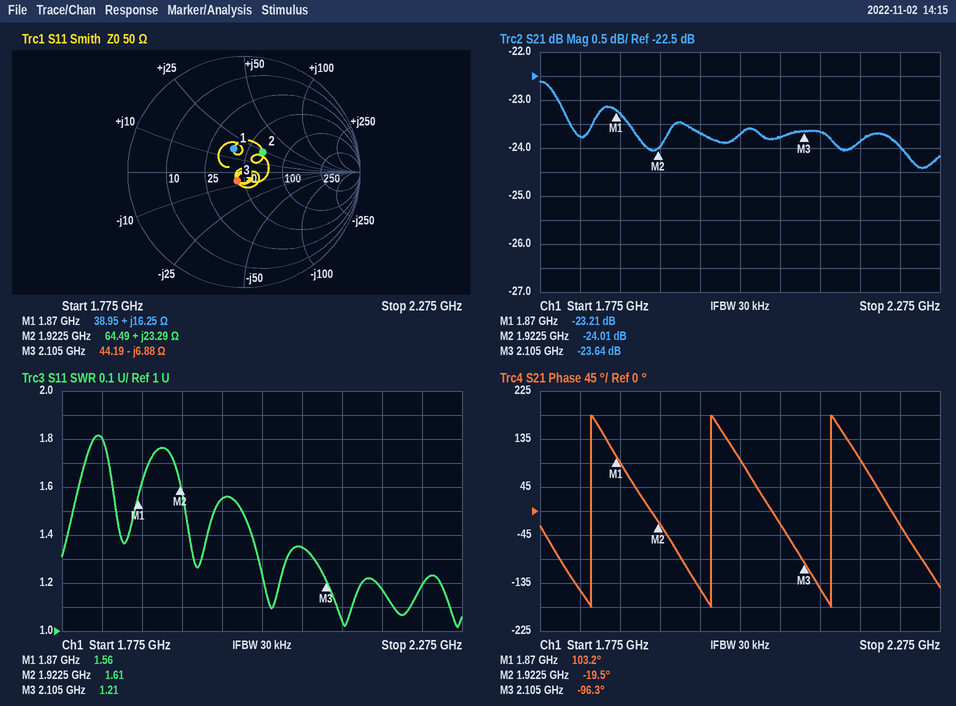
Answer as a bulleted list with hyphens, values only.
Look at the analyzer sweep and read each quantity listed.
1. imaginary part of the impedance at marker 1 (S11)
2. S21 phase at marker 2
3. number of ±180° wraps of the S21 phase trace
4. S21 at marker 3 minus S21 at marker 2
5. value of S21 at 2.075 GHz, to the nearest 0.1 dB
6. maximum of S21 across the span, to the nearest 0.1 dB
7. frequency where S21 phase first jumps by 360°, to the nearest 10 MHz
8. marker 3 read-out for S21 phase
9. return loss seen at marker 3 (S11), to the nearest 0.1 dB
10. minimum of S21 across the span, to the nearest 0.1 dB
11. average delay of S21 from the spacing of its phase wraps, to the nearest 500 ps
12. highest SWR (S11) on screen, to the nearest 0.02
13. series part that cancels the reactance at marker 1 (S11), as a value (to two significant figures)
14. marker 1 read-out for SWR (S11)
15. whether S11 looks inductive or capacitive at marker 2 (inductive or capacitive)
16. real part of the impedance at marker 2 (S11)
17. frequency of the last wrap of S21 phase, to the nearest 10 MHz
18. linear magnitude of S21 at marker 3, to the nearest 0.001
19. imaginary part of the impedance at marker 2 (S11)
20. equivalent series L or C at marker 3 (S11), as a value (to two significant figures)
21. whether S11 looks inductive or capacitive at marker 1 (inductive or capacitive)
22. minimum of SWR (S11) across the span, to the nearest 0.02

- +16.25 Ω
- -19.5°
- 3
- 0.37 dB
- -23.8 dB
- -22.6 dB
- 1.84 GHz
- -96.3°
- 20.4 dB
- -24.4 dB
- 6.5 ns
- 1.82
- 5.2 pF
- 1.56
- inductive
- 64.49 Ω
- 2.14 GHz
- 0.066
- +23.29 Ω
- 11 pF
- inductive
- 1.02
